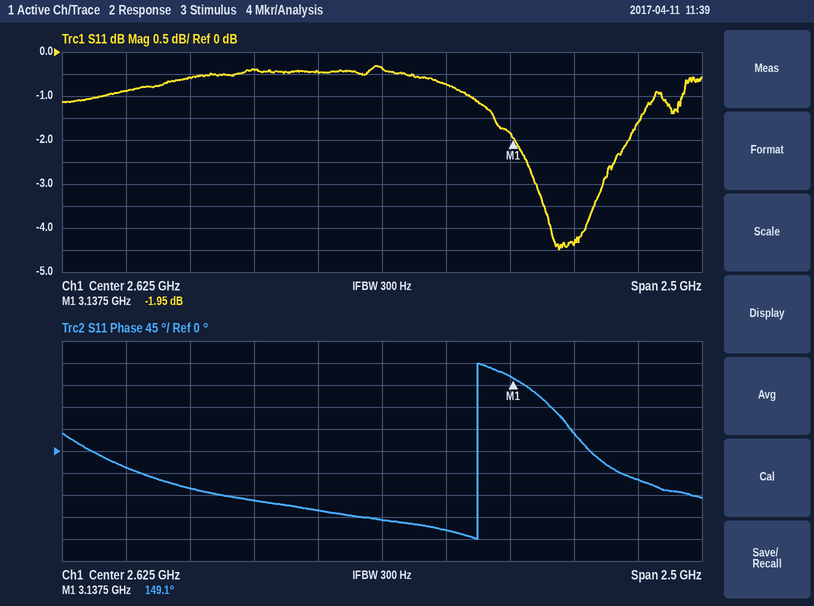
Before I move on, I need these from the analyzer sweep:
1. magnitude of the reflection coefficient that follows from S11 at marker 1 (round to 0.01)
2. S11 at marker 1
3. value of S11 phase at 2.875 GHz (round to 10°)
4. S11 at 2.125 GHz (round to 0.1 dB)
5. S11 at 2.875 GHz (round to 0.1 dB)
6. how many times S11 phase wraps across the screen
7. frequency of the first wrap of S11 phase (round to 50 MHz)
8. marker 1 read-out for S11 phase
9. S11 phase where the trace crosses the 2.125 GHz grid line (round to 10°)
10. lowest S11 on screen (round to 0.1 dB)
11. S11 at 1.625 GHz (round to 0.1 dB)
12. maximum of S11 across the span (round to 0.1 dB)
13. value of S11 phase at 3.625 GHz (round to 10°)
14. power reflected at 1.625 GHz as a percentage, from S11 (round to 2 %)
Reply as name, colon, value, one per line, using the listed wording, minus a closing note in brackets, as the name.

magnitude of the reflection coefficient that follows from S11 at marker 1: 0.80
S11 at marker 1: -1.95 dB
value of S11 phase at 2.875 GHz: -160°
S11 at 2.125 GHz: -0.4 dB
S11 at 2.875 GHz: -0.7 dB
how many times S11 phase wraps across the screen: 1
frequency of the first wrap of S11 phase: 3.00 GHz
marker 1 read-out for S11 phase: 149.1°
S11 phase where the trace crosses the 2.125 GHz grid line: -100°
lowest S11 on screen: -4.5 dB
S11 at 1.625 GHz: -0.9 dB
maximum of S11 across the span: -0.3 dB
value of S11 phase at 3.625 GHz: -60°
power reflected at 1.625 GHz as a percentage, from S11: 82 %
